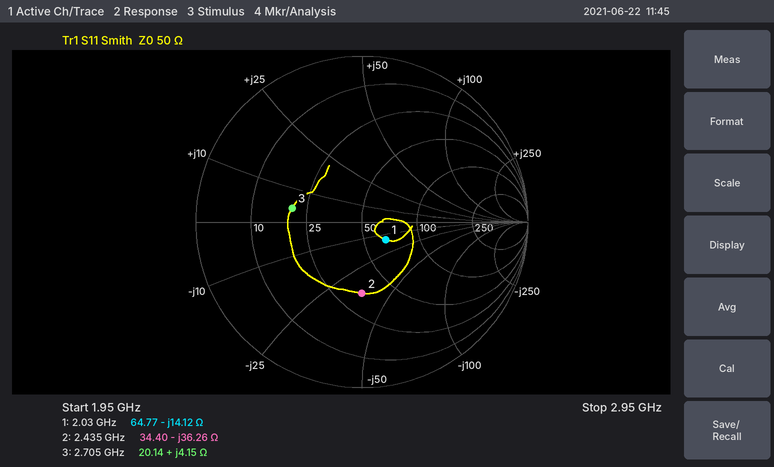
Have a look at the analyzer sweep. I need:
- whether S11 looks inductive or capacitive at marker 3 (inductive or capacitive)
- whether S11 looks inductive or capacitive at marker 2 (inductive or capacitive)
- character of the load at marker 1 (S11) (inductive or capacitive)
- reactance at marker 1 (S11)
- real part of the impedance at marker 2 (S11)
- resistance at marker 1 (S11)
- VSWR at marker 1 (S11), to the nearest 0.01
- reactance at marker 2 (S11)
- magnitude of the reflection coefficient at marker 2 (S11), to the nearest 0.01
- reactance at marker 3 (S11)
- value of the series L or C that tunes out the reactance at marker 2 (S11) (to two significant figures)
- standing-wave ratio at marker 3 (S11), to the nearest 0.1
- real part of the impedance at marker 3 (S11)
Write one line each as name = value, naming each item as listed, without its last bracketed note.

whether S11 looks inductive or capacitive at marker 3 = inductive
whether S11 looks inductive or capacitive at marker 2 = capacitive
character of the load at marker 1 (S11) = capacitive
reactance at marker 1 = -14.12 Ω
real part of the impedance at marker 2 = 34.40 Ω
resistance at marker 1 = 64.77 Ω
VSWR at marker 1 (S11), to the nearest 0.01 = 1.43
reactance at marker 2 = -36.26 Ω
magnitude of the reflection coefficient at marker 2 (S11), to the nearest 0.01 = 0.43
reactance at marker 3 = +4.15 Ω
value of the series L or C that tunes out the reactance at marker 2 (S11) = 2.4 nH
standing-wave ratio at marker 3 (S11), to the nearest 0.1 = 2.5
real part of the impedance at marker 3 = 20.14 Ω
